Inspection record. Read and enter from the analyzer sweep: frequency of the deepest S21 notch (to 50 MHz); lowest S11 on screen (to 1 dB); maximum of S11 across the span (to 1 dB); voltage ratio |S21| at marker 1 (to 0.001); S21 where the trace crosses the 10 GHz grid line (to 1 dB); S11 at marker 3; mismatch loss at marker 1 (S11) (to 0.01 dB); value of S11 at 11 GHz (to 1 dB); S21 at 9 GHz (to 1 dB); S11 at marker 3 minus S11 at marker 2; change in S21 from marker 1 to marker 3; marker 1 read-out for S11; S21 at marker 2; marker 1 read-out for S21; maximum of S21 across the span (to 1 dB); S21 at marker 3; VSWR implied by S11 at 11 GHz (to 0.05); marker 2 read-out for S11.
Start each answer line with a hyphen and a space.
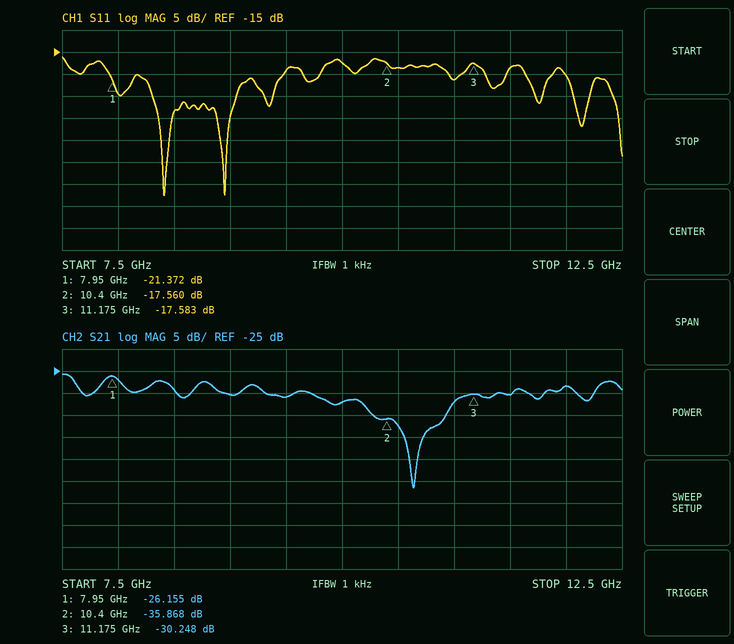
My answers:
- 10.65 GHz
- -48 dB
- -16 dB
- 0.049
- -32 dB
- -17.583 dB
- 0.03 dB
- -21 dB
- -30 dB
- -0.023 dB
- -4.093 dB
- -21.372 dB
- -35.868 dB
- -26.155 dB
- -26 dB
- -30.248 dB
- 1.20
- -17.560 dB
